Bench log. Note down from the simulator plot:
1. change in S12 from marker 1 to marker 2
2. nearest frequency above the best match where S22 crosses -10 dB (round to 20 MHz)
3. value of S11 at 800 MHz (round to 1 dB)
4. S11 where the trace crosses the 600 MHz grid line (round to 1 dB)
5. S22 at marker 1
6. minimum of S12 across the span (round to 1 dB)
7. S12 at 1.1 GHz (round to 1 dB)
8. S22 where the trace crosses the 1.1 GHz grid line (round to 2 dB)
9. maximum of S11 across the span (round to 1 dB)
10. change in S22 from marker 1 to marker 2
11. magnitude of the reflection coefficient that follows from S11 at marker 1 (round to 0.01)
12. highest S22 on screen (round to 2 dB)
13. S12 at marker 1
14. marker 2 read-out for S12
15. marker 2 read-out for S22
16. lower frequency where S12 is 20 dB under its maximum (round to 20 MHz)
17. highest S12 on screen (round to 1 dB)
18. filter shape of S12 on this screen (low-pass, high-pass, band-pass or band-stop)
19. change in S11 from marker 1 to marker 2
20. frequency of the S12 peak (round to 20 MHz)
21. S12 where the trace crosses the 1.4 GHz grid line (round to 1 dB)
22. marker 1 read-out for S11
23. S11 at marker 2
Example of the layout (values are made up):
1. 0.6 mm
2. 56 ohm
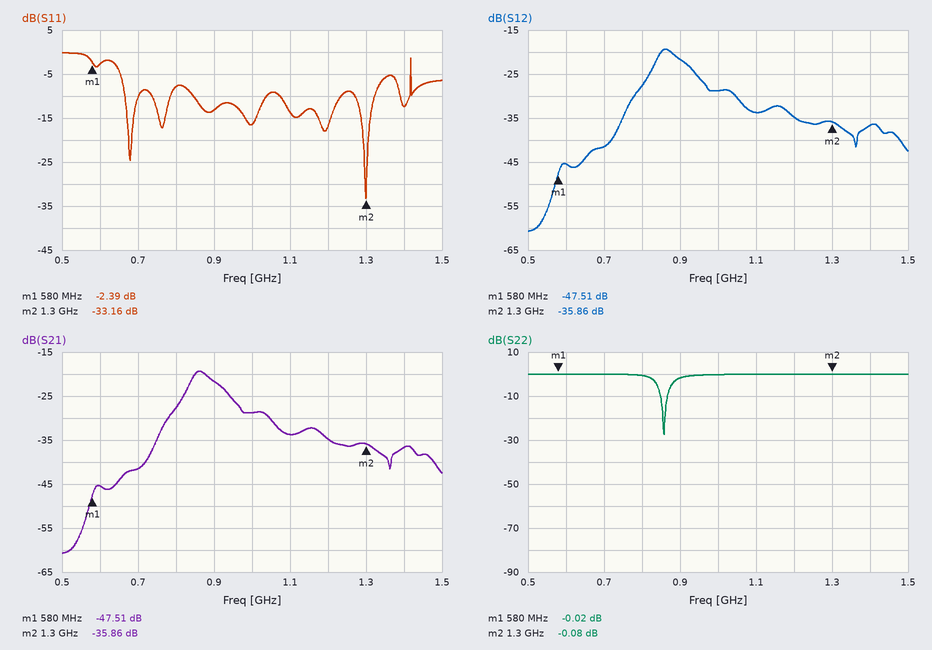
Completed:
1. 11.65 dB
2. 860 MHz
3. -8 dB
4. -3 dB
5. -0.02 dB
6. -61 dB
7. -34 dB
8. 0 dB
9. 0 dB
10. -0.06 dB
11. 0.76
12. 0 dB
13. -47.51 dB
14. -35.86 dB
15. -0.08 dB
16. 720 MHz
17. -19 dB
18. band-pass
19. -30.77 dB
20. 860 MHz
21. -37 dB
22. -2.39 dB
23. -33.16 dB
